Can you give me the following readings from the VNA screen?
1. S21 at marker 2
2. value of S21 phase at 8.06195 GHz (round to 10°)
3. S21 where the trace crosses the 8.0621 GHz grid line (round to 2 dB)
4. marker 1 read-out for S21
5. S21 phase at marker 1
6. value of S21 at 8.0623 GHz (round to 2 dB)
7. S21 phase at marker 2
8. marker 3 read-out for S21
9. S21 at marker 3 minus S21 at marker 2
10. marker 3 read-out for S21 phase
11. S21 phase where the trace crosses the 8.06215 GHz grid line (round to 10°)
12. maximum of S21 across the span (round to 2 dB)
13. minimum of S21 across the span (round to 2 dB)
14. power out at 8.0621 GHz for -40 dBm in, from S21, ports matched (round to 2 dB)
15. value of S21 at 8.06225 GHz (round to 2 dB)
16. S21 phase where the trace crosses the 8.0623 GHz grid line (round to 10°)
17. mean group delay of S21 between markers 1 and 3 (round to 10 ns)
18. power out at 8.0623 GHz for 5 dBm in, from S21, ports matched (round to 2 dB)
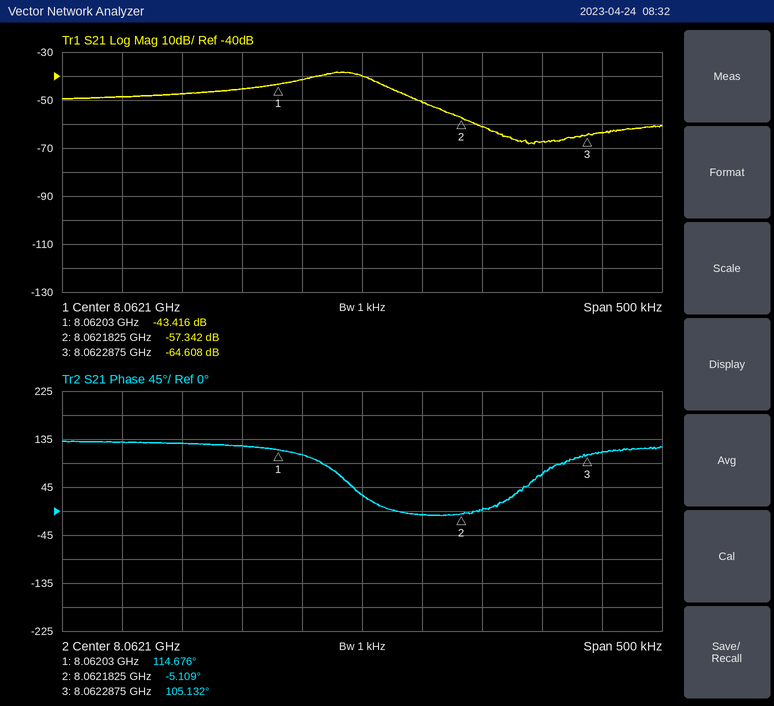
-57.342 dB
130°
-40 dB
-43.416 dB
114.676°
-64 dB
-5.109°
-64.608 dB
-7.266 dB
105.132°
-10°
-38 dB
-68 dB
-80 dBm
-68 dB
110°
100 ns
-58 dBm
